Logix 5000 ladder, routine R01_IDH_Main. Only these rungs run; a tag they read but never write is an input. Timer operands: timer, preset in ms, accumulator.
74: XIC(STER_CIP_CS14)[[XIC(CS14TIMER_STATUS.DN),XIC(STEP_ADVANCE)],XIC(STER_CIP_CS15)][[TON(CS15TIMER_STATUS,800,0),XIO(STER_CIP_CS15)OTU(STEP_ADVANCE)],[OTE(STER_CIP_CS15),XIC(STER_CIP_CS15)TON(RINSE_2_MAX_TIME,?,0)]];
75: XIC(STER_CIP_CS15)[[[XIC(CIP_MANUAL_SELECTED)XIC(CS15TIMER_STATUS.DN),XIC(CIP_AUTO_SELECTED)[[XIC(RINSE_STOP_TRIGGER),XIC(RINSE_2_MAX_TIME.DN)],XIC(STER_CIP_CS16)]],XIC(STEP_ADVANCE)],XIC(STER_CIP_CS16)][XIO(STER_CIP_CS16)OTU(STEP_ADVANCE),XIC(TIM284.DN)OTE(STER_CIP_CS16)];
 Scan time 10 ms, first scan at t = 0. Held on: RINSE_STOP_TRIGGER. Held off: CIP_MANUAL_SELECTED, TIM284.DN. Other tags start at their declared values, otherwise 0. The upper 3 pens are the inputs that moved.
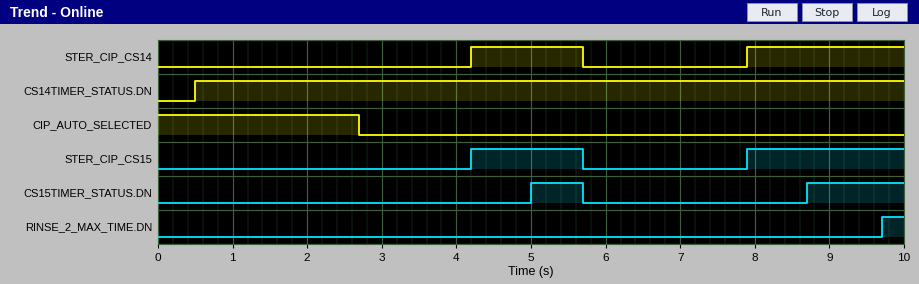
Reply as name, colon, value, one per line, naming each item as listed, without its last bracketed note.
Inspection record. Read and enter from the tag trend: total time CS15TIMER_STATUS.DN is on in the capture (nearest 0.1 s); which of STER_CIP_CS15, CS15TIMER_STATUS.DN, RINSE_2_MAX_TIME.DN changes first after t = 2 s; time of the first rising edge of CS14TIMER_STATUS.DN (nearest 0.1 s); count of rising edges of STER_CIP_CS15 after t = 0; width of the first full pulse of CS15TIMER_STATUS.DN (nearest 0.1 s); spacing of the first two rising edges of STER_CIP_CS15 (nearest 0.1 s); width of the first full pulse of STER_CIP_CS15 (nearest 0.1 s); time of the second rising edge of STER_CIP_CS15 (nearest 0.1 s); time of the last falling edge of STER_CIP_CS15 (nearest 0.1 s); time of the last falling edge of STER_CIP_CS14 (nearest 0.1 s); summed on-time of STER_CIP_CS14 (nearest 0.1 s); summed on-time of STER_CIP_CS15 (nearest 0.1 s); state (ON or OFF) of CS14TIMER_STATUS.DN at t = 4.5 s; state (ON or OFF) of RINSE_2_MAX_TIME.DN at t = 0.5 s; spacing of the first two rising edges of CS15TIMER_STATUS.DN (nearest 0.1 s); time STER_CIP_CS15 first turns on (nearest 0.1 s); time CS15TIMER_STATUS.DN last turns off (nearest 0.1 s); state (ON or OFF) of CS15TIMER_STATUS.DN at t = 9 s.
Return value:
total time CS15TIMER_STATUS.DN is on in the capture: 2.0 s
which of STER_CIP_CS15, CS15TIMER_STATUS.DN, RINSE_2_MAX_TIME.DN changes first after t = 2 s: STER_CIP_CS15
time of the first rising edge of CS14TIMER_STATUS.DN: 0.5 s
count of rising edges of STER_CIP_CS15 after t = 0: 2
width of the first full pulse of CS15TIMER_STATUS.DN: 0.7 s
spacing of the first two rising edges of STER_CIP_CS15: 3.7 s
width of the first full pulse of STER_CIP_CS15: 1.5 s
time of the second rising edge of STER_CIP_CS15: 7.9 s
time of the last falling edge of STER_CIP_CS15: 5.7 s
time of the last falling edge of STER_CIP_CS14: 5.7 s
summed on-time of STER_CIP_CS14: 3.6 s
summed on-time of STER_CIP_CS15: 3.6 s
state (ON or OFF) of CS14TIMER_STATUS.DN at t = 4.5 s: ON
state (ON or OFF) of RINSE_2_MAX_TIME.DN at t = 0.5 s: OFF
spacing of the first two rising edges of CS15TIMER_STATUS.DN: 3.7 s
time STER_CIP_CS15 first turns on: 4.2 s
time CS15TIMER_STATUS.DN last turns off: 5.7 s
state (ON or OFF) of CS15TIMER_STATUS.DN at t = 9 s: ON
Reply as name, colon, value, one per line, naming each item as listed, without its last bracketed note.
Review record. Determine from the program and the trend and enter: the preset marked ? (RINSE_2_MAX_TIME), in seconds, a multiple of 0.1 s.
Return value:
the preset marked ? (RINSE_2_MAX_TIME), in seconds, a multiple of 0.1 s: 1.8 s
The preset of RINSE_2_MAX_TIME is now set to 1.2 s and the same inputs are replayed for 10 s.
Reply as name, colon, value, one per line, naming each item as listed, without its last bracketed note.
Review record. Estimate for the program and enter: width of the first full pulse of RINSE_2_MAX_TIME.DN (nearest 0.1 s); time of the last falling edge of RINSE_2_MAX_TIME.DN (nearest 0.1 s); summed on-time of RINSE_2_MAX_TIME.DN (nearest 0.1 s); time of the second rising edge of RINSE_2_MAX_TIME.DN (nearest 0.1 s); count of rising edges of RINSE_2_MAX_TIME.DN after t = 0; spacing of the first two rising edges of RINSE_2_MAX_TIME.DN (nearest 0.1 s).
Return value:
width of the first full pulse of RINSE_2_MAX_TIME.DN: 0.3 s
time of the last falling edge of RINSE_2_MAX_TIME.DN: 5.7 s
summed on-time of RINSE_2_MAX_TIME.DN: 1.2 s
time of the second rising edge of RINSE_2_MAX_TIME.DN: 9.1 s
count of rising edges of RINSE_2_MAX_TIME.DN after t = 0: 2
spacing of the first two rising edges of RINSE_2_MAX_TIME.DN: 3.7 s
